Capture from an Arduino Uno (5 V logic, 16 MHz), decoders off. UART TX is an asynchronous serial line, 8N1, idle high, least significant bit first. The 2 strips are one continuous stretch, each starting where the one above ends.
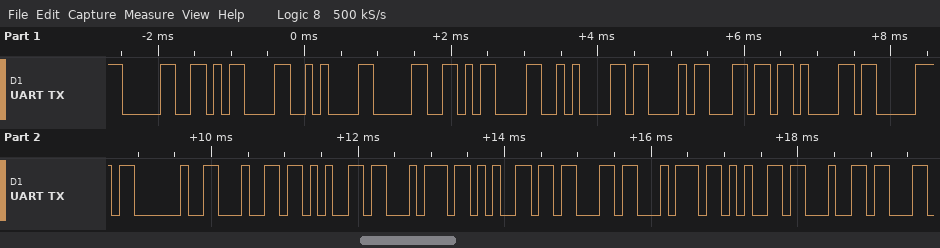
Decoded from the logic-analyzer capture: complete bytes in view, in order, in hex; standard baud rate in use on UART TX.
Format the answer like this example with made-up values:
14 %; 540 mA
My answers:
0x30 0x0D 0x0A 0x30 0x0D 0x0A 0x43 0x6C 0x61 0x70 0x20 0x64 0x65 0x74 0x65 0x63 0x74 0x65 0x64; 9600 baud
